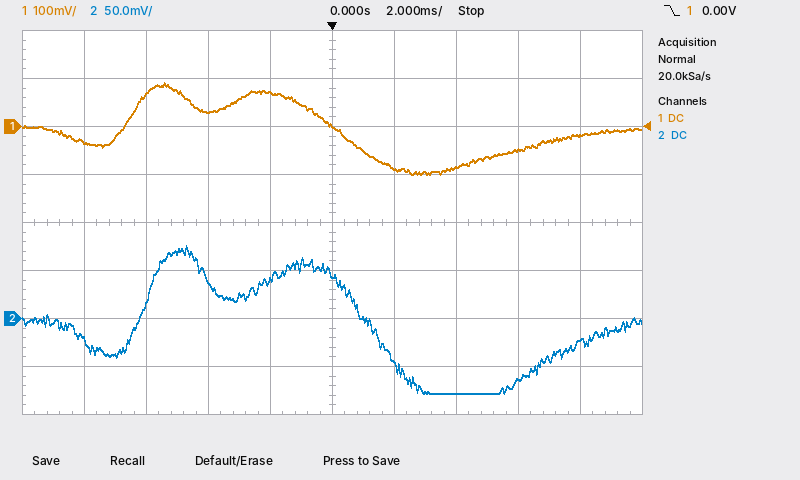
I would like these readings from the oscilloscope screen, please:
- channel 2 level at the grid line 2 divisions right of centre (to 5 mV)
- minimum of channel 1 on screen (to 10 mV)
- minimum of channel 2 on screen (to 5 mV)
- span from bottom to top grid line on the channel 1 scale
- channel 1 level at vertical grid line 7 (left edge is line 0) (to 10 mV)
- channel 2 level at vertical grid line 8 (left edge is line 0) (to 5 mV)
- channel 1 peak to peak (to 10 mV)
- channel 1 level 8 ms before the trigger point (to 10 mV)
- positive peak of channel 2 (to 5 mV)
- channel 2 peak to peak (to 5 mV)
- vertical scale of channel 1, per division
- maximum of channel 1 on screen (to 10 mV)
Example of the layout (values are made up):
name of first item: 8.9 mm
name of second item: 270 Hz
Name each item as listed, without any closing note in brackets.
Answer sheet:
channel 2 level at the grid line 2 divisions right of centre: -80 mV
minimum of channel 1 on screen: -100 mV
minimum of channel 2 on screen: -80 mV
span from bottom to top grid line on the channel 1 scale: 800 mV
channel 1 level at vertical grid line 7 (left edge is line 0): -90 mV
channel 2 level at vertical grid line 8 (left edge is line 0): -65 mV
channel 1 peak to peak: 190 mV
channel 1 level 8 ms before the trigger point: -30 mV
positive peak of channel 2: 75 mV
channel 2 peak to peak: 155 mV
vertical scale of channel 1, per division: 100 mV
maximum of channel 1 on screen: 90 mV
